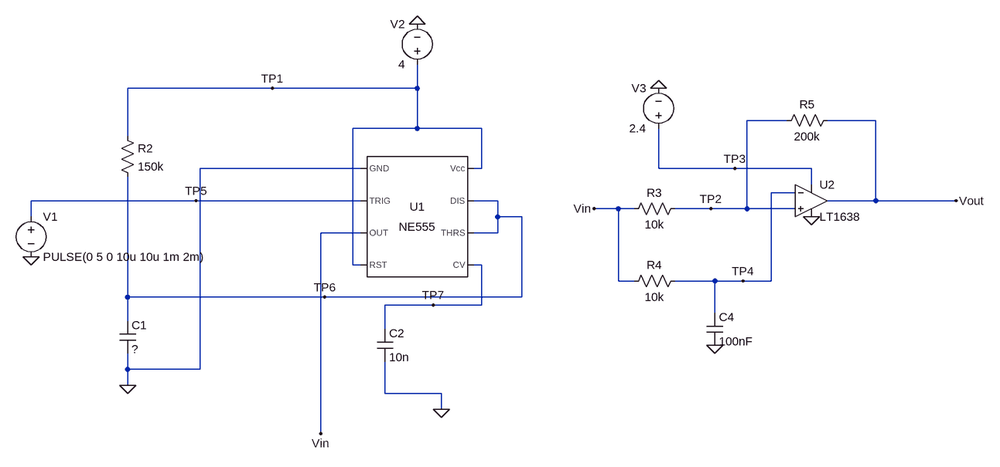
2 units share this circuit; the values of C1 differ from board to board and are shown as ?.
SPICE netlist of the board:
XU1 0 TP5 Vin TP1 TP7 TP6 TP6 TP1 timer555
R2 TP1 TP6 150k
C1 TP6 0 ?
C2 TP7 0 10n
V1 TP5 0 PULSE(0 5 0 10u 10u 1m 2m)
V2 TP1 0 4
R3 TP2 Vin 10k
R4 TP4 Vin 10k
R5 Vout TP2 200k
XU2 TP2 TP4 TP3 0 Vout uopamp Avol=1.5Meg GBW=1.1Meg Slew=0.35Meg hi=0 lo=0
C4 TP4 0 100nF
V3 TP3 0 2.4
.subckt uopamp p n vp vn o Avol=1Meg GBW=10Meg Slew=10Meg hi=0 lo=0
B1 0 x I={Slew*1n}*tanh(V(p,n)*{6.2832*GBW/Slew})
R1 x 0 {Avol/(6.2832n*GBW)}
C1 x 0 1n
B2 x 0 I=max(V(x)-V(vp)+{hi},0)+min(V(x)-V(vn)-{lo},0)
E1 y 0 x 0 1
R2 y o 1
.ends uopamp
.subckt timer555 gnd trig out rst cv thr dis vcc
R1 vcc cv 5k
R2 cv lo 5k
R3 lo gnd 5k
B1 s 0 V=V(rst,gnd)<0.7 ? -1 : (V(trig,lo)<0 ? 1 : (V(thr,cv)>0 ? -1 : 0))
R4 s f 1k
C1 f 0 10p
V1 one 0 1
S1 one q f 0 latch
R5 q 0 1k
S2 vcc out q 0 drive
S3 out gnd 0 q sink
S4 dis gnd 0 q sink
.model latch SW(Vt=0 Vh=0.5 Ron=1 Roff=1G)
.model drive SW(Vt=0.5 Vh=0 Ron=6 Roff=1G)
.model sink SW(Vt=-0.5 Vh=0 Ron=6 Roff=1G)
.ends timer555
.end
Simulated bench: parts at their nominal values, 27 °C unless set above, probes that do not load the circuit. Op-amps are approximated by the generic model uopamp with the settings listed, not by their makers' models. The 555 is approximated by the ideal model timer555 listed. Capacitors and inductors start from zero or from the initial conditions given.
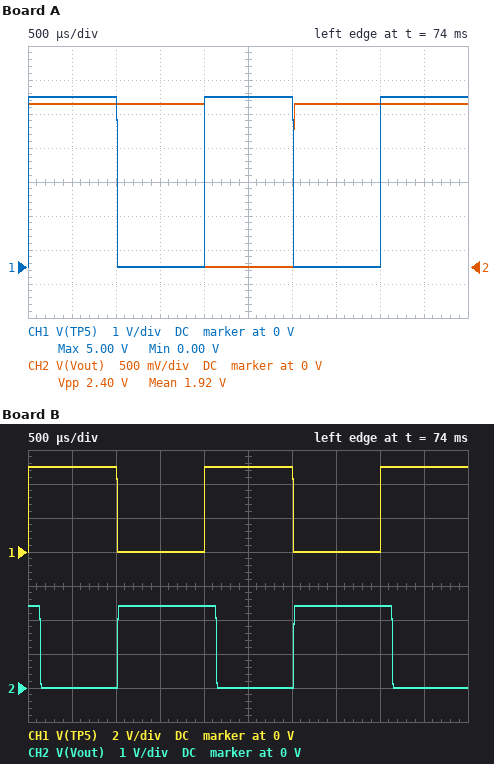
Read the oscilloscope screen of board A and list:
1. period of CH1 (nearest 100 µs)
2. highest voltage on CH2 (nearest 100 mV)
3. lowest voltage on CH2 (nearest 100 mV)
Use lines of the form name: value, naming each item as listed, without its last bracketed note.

period of CH1: 2.0 ms
highest voltage on CH2: 2.4 V
lowest voltage on CH2: 0 V
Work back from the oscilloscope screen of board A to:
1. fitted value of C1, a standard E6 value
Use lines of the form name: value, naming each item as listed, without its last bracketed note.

fitted value of C1, a standard E6 value: 15 nF
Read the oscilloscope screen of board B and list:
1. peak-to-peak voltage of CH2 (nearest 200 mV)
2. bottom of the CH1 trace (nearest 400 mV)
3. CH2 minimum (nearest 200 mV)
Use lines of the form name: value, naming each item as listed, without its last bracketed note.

peak-to-peak voltage of CH2: 2.4 V
bottom of the CH1 trace: 0 V
CH2 minimum: 0 V
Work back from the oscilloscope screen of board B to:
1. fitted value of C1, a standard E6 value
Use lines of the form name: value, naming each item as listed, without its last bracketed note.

fitted value of C1, a standard E6 value: 6.8 nF
